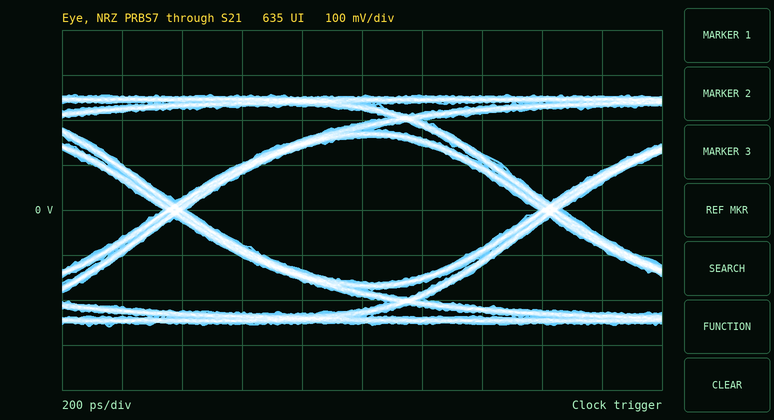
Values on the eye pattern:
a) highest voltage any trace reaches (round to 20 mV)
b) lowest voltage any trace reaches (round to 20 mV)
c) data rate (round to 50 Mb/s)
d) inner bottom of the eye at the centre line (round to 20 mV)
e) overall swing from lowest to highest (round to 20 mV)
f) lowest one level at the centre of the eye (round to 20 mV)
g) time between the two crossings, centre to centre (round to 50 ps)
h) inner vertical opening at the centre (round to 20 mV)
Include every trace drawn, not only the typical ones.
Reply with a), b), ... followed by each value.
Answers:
a) 260 mV
b) -260 mV
c) 800 Mb/s
d) -160 mV
e) 520 mV
f) 160 mV
g) 1.25 ns
h) 320 mV
